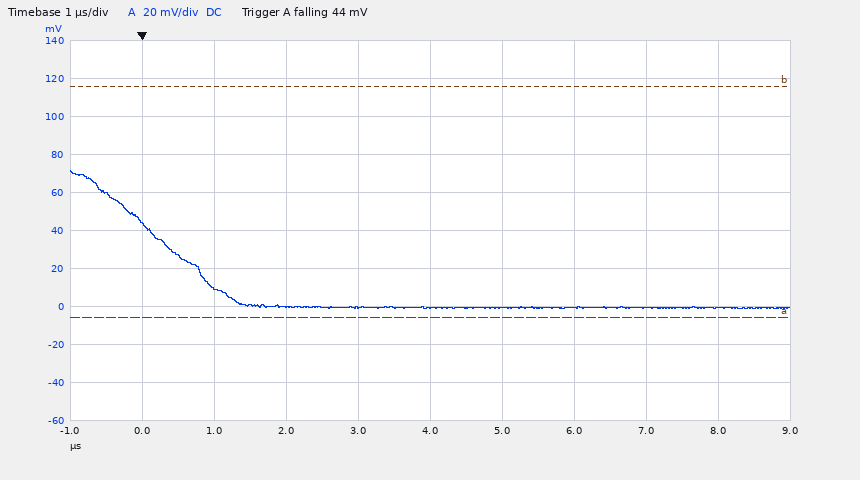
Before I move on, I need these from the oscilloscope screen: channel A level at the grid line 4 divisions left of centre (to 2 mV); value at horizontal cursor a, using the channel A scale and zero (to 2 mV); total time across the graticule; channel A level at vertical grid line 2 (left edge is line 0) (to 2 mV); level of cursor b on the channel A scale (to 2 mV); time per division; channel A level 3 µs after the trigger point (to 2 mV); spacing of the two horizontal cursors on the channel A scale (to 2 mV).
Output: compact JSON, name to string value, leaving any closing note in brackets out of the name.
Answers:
{"channel A level at the grid line 4 divisions left of centre": "44 mV", "value at horizontal cursor a, using the channel A scale and zero": "-6 mV", "total time across the graticule": "10 µs", "channel A level at vertical grid line 2 (left edge is line 0)": "10 mV", "level of cursor b on the channel A scale": "116 mV", "time per division": "1 µs", "channel A level 3 µs after the trigger point": "0 mV", "spacing of the two horizontal cursors on the channel A scale": "122 mV"}
